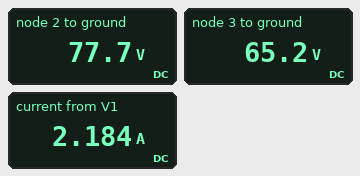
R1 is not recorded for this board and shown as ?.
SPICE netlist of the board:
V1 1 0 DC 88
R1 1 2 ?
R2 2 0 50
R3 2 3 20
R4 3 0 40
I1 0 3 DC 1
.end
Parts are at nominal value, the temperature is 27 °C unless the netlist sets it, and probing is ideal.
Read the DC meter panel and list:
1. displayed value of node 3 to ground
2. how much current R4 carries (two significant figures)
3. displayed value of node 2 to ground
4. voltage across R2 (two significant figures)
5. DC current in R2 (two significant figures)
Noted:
65.2 V
1.6 A
77.7 V
78 V
1.6 A
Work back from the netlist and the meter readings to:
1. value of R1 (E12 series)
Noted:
4.7 Ω
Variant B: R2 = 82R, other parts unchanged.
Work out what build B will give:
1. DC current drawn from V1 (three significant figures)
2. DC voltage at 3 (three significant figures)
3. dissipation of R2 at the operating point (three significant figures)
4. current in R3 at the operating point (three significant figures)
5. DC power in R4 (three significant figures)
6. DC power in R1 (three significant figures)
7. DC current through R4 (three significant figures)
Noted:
1.65 A
66.8 V
78.5 W
671 mA
112 W
12.8 W
1.67 A
